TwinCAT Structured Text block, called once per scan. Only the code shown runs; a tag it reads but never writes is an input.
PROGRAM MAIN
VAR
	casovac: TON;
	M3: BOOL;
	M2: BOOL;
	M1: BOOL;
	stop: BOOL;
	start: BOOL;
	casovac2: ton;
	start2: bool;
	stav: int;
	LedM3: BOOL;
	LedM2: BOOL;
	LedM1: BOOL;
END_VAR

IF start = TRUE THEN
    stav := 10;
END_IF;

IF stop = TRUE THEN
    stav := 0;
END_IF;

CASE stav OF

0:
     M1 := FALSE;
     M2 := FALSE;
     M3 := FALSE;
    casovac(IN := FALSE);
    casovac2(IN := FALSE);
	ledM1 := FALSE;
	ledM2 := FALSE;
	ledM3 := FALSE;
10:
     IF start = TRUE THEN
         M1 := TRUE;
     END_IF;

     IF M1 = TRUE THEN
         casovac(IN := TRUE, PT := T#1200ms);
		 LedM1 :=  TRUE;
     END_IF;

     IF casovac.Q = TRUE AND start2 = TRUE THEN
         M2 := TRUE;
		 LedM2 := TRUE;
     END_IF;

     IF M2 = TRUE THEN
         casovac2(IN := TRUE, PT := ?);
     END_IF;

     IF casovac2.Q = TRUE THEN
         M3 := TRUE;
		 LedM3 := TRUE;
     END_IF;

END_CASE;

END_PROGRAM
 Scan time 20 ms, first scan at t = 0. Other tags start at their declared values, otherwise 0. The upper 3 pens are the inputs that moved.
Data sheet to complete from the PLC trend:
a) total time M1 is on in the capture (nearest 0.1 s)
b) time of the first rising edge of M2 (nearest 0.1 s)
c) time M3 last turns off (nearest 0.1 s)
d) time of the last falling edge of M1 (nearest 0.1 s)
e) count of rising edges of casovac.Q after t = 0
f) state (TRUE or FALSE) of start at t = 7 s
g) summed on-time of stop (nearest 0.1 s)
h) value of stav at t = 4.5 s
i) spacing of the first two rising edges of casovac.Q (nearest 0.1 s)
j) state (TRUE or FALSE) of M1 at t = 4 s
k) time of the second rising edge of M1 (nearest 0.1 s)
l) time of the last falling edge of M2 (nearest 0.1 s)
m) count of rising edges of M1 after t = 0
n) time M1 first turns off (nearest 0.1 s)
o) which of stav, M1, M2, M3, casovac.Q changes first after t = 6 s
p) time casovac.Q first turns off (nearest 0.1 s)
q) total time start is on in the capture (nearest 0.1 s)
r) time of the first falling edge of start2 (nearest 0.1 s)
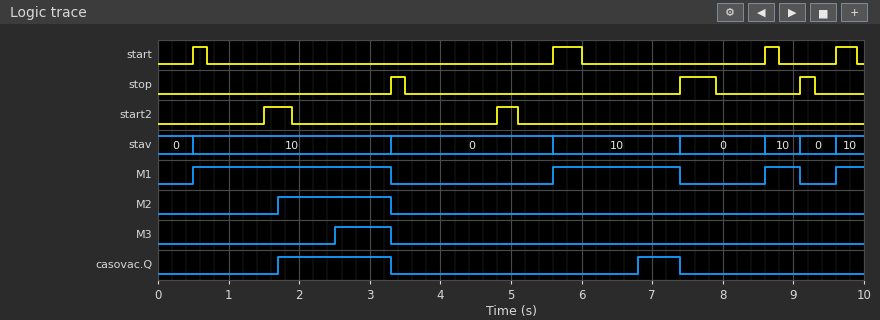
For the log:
5.5 s
1.7 s
3.3 s
9.1 s
2
FALSE
0.9 s
0
5.1 s
FALSE
5.6 s
3.3 s
4
3.3 s
casovac.Q
3.3 s
1.1 s
1.9 s
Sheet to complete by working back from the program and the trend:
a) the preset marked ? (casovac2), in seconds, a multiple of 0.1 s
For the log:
0.8 s
